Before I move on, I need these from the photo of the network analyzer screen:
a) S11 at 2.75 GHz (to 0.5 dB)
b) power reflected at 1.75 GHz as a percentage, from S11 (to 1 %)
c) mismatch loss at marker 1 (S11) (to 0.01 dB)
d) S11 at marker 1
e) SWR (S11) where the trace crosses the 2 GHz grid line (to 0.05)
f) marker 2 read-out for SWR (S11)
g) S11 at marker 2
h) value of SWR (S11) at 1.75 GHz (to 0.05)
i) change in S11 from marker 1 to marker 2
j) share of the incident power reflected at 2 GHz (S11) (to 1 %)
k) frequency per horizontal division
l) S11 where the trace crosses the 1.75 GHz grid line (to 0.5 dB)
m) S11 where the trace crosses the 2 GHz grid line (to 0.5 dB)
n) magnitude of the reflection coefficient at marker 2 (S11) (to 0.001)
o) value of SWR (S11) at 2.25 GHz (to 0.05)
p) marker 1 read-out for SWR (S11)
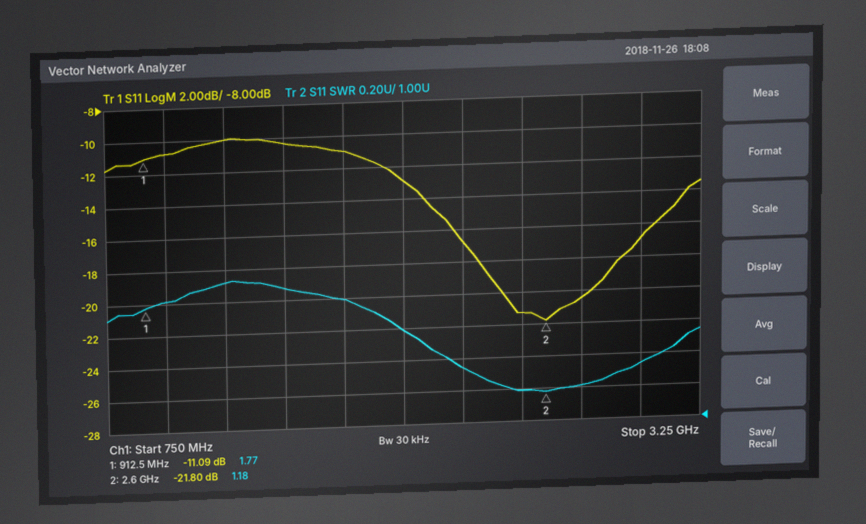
-20.5 dB
8 %
0.35 dB
-11.09 dB
1.60
1.18
-21.80 dB
1.80
-10.71 dB
5 %
250 MHz
-11.0 dB
-13.0 dB
0.081
1.35
1.77
